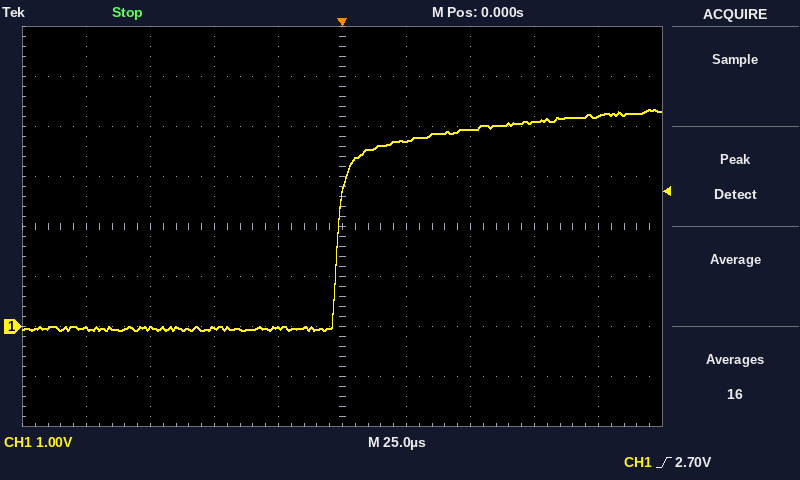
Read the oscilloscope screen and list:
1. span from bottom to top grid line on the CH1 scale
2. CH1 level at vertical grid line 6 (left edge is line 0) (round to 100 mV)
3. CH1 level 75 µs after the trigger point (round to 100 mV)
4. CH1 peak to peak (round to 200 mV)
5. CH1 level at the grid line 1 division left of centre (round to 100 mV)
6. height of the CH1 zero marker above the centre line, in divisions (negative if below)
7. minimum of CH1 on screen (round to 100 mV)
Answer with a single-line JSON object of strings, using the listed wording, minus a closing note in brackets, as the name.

{"span from bottom to top grid line on the CH1 scale": "8 V", "CH1 level at vertical grid line 6 (left edge is line 0)": "3.7 V", "CH1 level 75 µs after the trigger point": "4.1 V", "CH1 peak to peak": "4.4 V", "CH1 level at the grid line 1 division left of centre": "0.0 V", "height of the CH1 zero marker above the centre line, in divisions": "-2.0 div", "minimum of CH1 on screen": "-100 mV"}
